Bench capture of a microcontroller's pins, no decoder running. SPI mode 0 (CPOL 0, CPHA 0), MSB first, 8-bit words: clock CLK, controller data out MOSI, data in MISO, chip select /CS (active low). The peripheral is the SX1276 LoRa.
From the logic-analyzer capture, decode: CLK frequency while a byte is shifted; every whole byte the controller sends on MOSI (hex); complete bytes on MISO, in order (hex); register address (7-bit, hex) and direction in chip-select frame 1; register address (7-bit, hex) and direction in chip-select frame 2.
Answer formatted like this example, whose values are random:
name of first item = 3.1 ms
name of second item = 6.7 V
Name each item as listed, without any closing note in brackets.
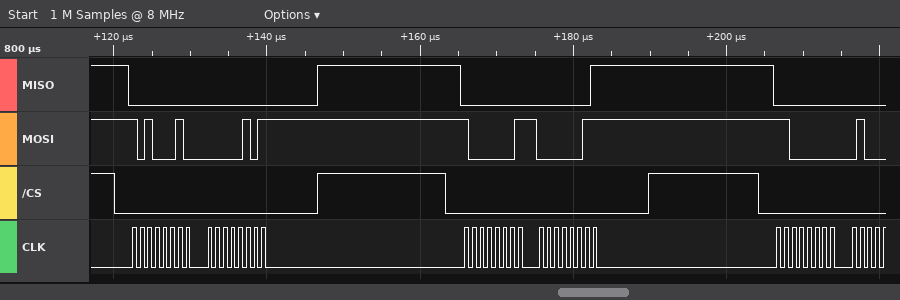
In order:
CLK frequency while a byte is shifted = 1 MHz
every whole byte the controller sends on MOSI = A2 05 81 03 C0
complete bytes on MISO, in order = 00 00 00 01 00
register address (7-bit, hex) and direction in chip-select frame 1 = 0x22 write
register address (7-bit, hex) and direction in chip-select frame 2 = 0x01 write
